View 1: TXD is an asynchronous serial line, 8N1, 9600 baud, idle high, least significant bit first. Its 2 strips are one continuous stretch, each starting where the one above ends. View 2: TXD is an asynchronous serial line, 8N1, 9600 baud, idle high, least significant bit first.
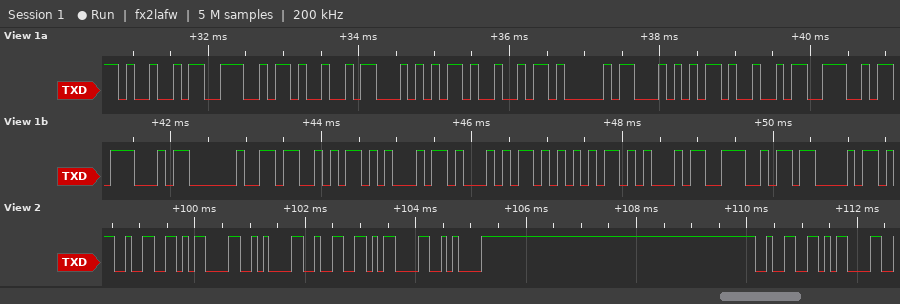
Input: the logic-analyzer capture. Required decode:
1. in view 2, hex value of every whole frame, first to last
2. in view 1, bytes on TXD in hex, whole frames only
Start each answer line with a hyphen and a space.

- 0x32 0x0D 0x0A 0x32 0x0D 0x0A 0x32 0x0D
- 49 4E 49 54 49 41 54 49 4E 47 20 53 45 51 55 45 4E 43
